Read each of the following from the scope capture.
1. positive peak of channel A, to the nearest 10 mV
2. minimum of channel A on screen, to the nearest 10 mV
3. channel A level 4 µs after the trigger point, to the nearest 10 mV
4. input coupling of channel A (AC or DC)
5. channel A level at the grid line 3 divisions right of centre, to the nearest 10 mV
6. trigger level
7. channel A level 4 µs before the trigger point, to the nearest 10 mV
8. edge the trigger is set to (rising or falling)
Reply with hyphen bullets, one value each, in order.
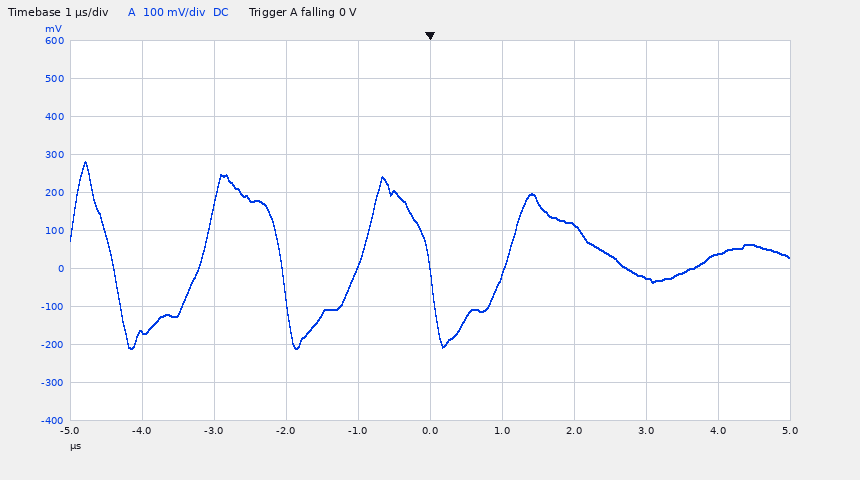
- 280 mV
- -210 mV
- 40 mV
- DC
- -20 mV
- 0 V
- -170 mV
- falling
